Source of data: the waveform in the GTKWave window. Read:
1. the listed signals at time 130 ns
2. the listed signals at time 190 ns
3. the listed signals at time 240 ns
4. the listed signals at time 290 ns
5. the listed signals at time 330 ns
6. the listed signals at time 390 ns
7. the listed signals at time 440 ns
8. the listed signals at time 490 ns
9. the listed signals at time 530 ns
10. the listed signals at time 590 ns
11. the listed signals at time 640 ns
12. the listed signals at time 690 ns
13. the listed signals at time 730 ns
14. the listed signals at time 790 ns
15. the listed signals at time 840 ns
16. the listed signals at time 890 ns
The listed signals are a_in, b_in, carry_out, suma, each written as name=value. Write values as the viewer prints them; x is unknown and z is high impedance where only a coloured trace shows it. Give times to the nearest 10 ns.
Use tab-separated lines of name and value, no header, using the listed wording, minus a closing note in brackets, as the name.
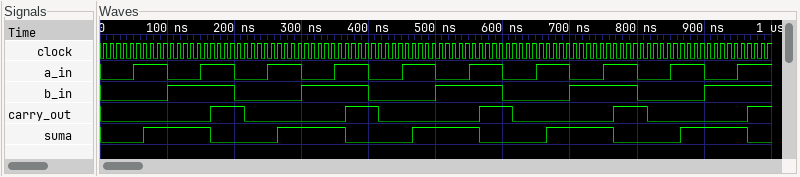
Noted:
the listed signals at time 130 ns	a_in=0, b_in=1, carry_out=0, suma=1
the listed signals at time 190 ns	a_in=1, b_in=1, carry_out=1, suma=0
the listed signals at time 240 ns	a_in=0, b_in=0, carry_out=0, suma=0
the listed signals at time 290 ns	a_in=1, b_in=0, carry_out=0, suma=1
the listed signals at time 330 ns	a_in=0, b_in=1, carry_out=0, suma=1
the listed signals at time 390 ns	a_in=1, b_in=1, carry_out=1, suma=0
the listed signals at time 440 ns	a_in=0, b_in=0, carry_out=0, suma=0
the listed signals at time 490 ns	a_in=1, b_in=0, carry_out=0, suma=1
the listed signals at time 530 ns	a_in=0, b_in=1, carry_out=0, suma=1
the listed signals at time 590 ns	a_in=1, b_in=1, carry_out=1, suma=0
the listed signals at time 640 ns	a_in=0, b_in=0, carry_out=0, suma=0
the listed signals at time 690 ns	a_in=1, b_in=0, carry_out=0, suma=1
the listed signals at time 730 ns	a_in=0, b_in=1, carry_out=0, suma=1
the listed signals at time 790 ns	a_in=1, b_in=1, carry_out=1, suma=0
the listed signals at time 840 ns	a_in=0, b_in=0, carry_out=0, suma=0
the listed signals at time 890 ns	a_in=1, b_in=0, carry_out=0, suma=1
